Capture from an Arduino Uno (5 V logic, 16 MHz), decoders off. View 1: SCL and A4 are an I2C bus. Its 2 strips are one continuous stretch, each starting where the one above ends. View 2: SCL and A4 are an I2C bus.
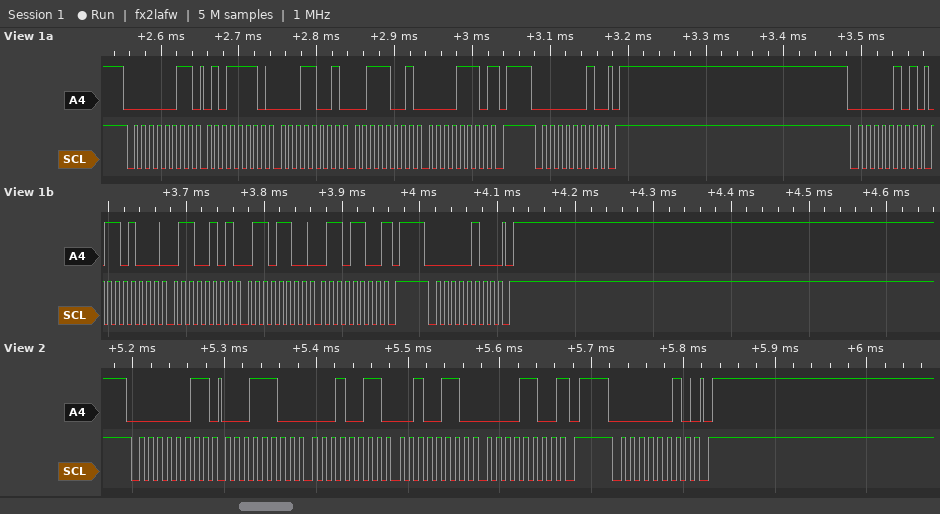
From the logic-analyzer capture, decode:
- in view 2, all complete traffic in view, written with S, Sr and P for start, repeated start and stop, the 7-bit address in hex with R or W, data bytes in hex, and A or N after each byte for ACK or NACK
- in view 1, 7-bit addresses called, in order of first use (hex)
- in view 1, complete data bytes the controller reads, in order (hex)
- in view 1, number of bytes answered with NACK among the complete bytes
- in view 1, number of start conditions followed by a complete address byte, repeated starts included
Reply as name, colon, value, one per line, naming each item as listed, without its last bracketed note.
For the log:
in view 2, all complete traffic in view, written with S, Sr and P for start, repeated start and stop, the 7-bit address in hex with R or W, data bytes in hex, and A or N after each byte for ACK or NACK: S 01R A 1C A 13 A 26 A 0C N P S 01W A P
in view 1, 7-bit addresses called, in order of first use: 0x01 0x02
in view 1, complete data bytes the controller reads, in order: 5E 19 39 0E 68 65 6C 6C
in view 1, number of bytes answered with NACK among the complete bytes: 2
in view 1, number of start conditions followed by a complete address byte, repeated starts included: 4
